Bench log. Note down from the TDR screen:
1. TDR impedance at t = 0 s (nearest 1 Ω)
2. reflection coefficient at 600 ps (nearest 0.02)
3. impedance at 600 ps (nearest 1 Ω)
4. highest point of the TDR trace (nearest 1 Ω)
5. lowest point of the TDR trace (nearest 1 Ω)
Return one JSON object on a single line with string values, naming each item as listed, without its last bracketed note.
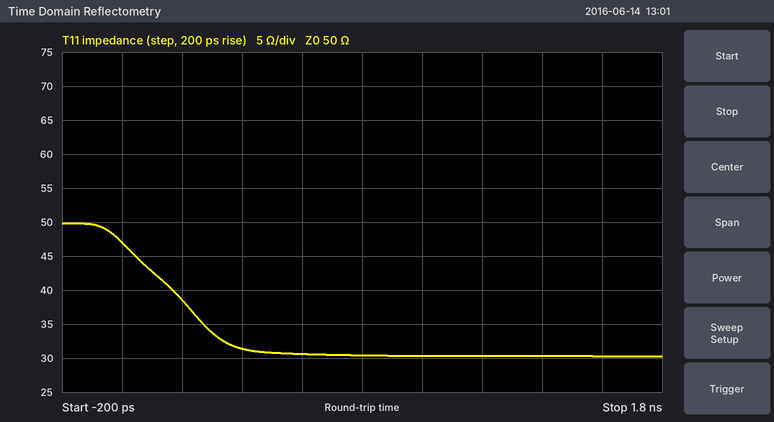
{"TDR impedance at t = 0 s": "47 Ω", "reflection coefficient at 600 ps": "-0.24", "impedance at 600 ps": "31 Ω", "highest point of the TDR trace": "50 Ω", "lowest point of the TDR trace": "30 Ω"}
